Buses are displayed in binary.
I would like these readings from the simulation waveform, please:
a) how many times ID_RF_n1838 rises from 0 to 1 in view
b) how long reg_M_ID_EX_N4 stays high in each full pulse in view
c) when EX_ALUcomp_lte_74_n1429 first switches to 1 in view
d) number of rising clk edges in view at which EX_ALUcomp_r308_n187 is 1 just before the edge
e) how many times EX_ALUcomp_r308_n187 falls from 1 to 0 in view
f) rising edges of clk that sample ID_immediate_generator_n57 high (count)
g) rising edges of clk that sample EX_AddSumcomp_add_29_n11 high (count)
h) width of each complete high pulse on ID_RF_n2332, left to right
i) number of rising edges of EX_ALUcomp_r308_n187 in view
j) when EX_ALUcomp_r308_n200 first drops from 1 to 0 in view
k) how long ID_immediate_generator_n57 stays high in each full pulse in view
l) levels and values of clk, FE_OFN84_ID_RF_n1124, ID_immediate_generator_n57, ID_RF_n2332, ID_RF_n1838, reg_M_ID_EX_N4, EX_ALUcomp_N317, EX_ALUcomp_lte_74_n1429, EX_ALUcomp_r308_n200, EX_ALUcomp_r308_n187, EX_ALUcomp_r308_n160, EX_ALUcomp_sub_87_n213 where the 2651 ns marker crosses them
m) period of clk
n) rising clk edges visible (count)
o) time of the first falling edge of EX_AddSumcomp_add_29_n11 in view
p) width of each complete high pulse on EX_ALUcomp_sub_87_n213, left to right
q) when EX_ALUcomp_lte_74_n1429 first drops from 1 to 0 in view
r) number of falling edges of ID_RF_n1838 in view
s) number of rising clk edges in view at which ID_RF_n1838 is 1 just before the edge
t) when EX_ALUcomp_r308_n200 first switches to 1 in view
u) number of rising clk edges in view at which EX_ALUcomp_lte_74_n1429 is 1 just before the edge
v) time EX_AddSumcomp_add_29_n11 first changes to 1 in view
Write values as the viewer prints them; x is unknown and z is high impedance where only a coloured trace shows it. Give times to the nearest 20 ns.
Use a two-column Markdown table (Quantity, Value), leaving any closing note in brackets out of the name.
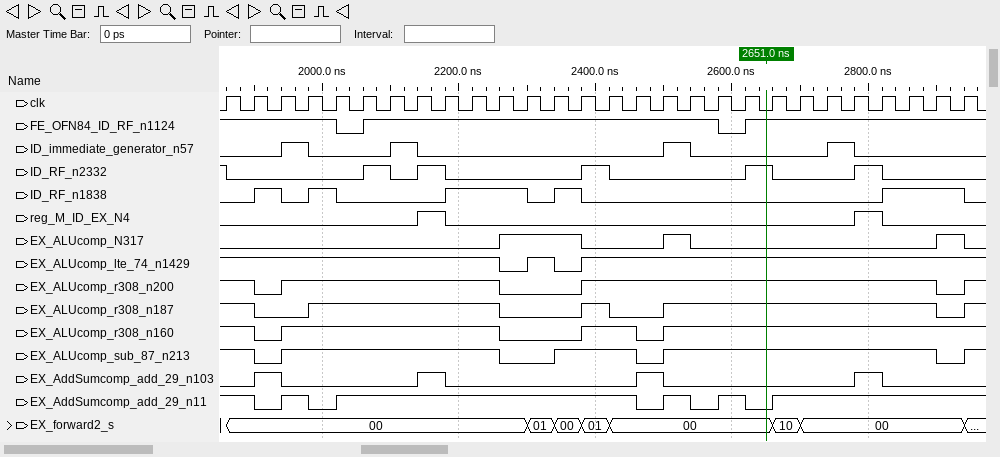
| Quantity | Value |
|---|---|
| how many times ID_RF_n1838 rises from 0 to 1 in view | 5 |
| how long reg_M_ID_EX_N4 stays high in each full pulse in view | 40 ns, 40 ns |
| when EX_ALUcomp_lte_74_n1429 first switches to 1 in view | 2300 ns |
| number of rising clk edges in view at which EX_ALUcomp_r308_n187 is 1 just before the edge | 20 |
| how many times EX_ALUcomp_r308_n187 falls from 1 to 0 in view | 4 |
| rising edges of clk that sample ID_immediate_generator_n57 high | 4 |
| rising edges of clk that sample EX_AddSumcomp_add_29_n11 high | 23 |
| width of each complete high pulse on ID_RF_n2332, left to right | 40 ns, 40 ns, 40 ns, 40 ns, 40 ns |
| number of rising edges of EX_ALUcomp_r308_n187 in view | 4 |
| when EX_ALUcomp_r308_n200 first drops from 1 to 0 in view | 1900 ns |
| how long ID_immediate_generator_n57 stays high in each full pulse in view | 40 ns, 40 ns, 40 ns, 40 ns |
| levels and values of clk, FE_OFN84_ID_RF_n1124, ID_immediate_generator_n57, ID_RF_n2332, ID_RF_n1838, reg_M_ID_EX_N4, EX_ALUcomp_N317, EX_ALUcomp_lte_74_n1429, EX_ALUcomp_r308_n200, EX_ALUcomp_r308_n187, EX_ALUcomp_r308_n160, EX_ALUcomp_sub_87_n213 where the 2651 ns marker crosses them | clk=0, FE_OFN84_ID_RF_n1124=1, ID_immediate_generator_n57=0, ID_RF_n2332=1, ID_RF_n1838=0, reg_M_ID_EX_N4=0, EX_ALUcomp_N317=0, EX_ALUcomp_lte_74_n1429=1, EX_ALUcomp_r308_n200=1, EX_ALUcomp_r308_n187=1, EX_ALUcomp_r308_n160=1, EX_ALUcomp_sub_87_n213=1 |
| period of clk | 40 ns |
| rising clk edges visible | 28 |
| time of the first falling edge of EX_AddSumcomp_add_29_n11 in view | 1900 ns |
| width of each complete high pulse on EX_ALUcomp_sub_87_n213, left to right | 320 ns, 120 ns, 400 ns |
| when EX_ALUcomp_lte_74_n1429 first drops from 1 to 0 in view | 2260 ns |
| number of falling edges of ID_RF_n1838 in view | 5 |
| number of rising clk edges in view at which ID_RF_n1838 is 1 just before the edge | 9 |
| when EX_ALUcomp_r308_n200 first switches to 1 in view | 1940 ns |
| number of rising clk edges in view at which EX_ALUcomp_lte_74_n1429 is 1 just before the edge | 26 |
| time EX_AddSumcomp_add_29_n11 first changes to 1 in view | 1940 ns |
